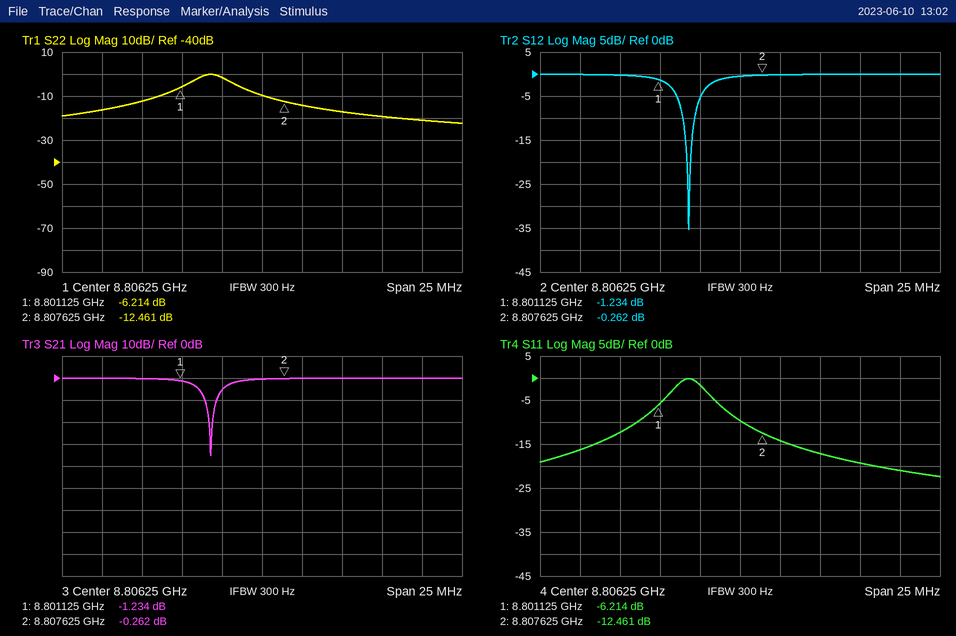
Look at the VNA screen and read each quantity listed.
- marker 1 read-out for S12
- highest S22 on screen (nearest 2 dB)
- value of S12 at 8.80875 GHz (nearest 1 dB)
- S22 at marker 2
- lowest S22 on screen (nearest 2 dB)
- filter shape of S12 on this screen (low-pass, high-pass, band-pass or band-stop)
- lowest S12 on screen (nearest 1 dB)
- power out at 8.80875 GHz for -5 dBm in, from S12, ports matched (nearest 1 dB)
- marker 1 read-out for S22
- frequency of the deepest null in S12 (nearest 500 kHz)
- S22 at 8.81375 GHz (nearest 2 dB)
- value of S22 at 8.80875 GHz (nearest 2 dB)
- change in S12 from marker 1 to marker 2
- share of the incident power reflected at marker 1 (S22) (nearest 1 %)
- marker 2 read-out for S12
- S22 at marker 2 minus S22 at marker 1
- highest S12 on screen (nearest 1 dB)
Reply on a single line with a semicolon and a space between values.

-1.234 dB; 0 dB; 0 dB; -12.461 dB; -22 dB; band-stop; -35 dB; -5 dBm; -6.214 dB; 8.8030 GHz; -20 dB; -14 dB; 0.972 dB; 24 %; -0.262 dB; -6.247 dB; 0 dB
